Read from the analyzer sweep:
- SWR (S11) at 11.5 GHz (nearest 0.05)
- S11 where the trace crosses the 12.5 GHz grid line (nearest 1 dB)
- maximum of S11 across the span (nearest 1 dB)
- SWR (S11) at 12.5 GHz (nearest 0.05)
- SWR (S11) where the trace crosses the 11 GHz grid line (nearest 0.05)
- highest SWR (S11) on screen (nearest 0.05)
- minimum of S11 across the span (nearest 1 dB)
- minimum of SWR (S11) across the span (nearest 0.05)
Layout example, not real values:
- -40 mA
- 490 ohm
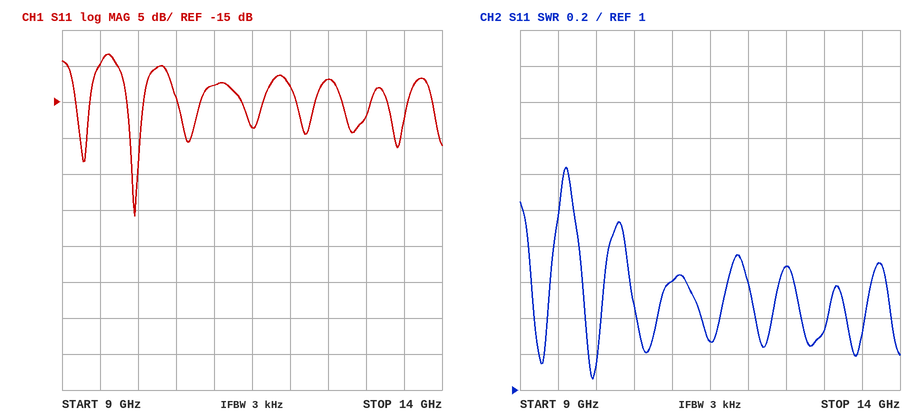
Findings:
- 1.25
- -12 dB
- -8 dB
- 1.70
- 1.60
- 2.25
- -31 dB
- 1.05
